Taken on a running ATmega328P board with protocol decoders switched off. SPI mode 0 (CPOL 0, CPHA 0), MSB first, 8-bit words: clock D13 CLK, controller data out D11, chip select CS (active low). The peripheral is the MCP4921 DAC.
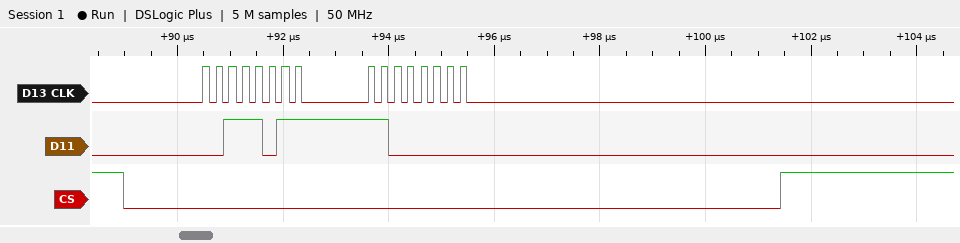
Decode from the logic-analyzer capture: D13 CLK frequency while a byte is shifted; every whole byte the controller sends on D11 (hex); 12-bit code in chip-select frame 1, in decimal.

4 MHz
3B C0
3008
